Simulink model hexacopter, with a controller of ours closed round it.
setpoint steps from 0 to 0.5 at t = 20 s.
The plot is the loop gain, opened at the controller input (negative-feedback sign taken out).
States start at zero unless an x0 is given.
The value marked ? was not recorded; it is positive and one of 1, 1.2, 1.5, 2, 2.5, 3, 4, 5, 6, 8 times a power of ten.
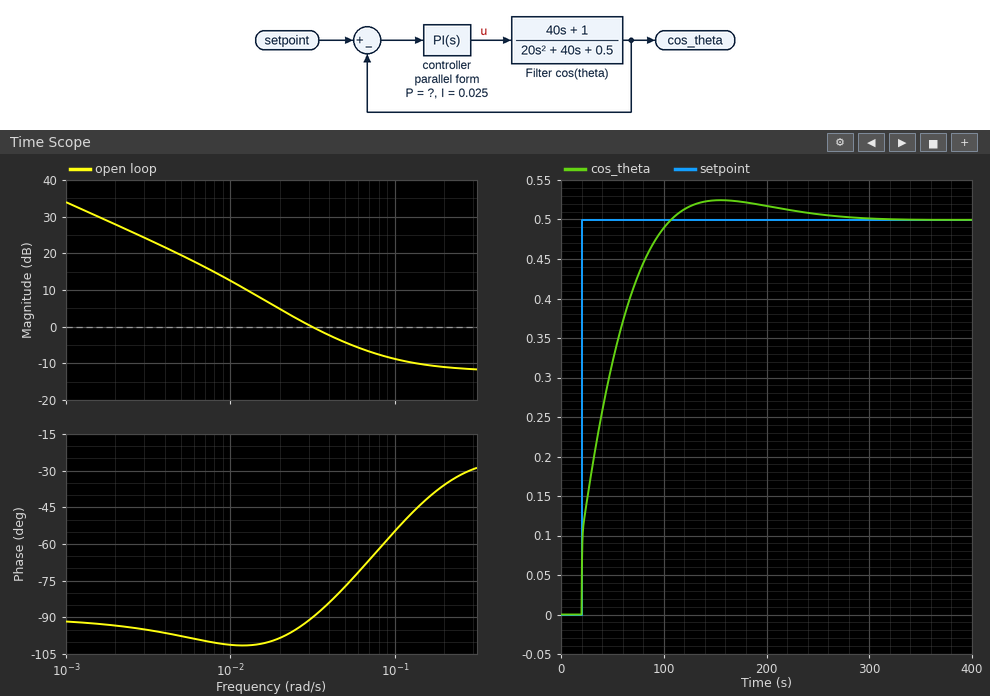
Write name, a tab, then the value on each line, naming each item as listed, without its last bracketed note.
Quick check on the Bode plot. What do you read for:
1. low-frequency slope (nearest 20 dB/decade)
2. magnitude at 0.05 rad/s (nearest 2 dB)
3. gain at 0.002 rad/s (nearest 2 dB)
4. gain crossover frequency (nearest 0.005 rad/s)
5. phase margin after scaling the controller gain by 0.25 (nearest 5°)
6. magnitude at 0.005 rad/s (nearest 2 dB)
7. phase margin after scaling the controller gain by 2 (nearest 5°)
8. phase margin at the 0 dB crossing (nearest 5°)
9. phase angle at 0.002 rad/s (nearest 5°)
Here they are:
low-frequency slope	-20 dB/decade
magnitude at 0.05 rad/s	-4 dB
gain at 0.002 rad/s	28 dB
gain crossover frequency	0.030 rad/s
phase margin after scaling the controller gain by 0.25	80°
magnitude at 0.005 rad/s	20 dB
phase margin after scaling the controller gain by 2	110°
phase margin at the 0 dB crossing	90°
phase angle at 0.002 rad/s	-95°
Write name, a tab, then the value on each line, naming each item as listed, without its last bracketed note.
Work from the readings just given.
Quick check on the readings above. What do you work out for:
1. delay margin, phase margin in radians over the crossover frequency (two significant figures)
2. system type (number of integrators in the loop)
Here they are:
delay margin, phase margin in radians over the crossover frequency	52 s
system type	1
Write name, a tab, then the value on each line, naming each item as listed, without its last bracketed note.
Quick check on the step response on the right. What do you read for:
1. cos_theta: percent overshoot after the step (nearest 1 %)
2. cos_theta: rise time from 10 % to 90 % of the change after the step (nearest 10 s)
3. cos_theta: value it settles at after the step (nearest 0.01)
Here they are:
cos_theta: percent overshoot after the step	5 %
cos_theta: rise time from 10 % to 90 % of the change after the step	60 s
cos_theta: value it settles at after the step	0.50
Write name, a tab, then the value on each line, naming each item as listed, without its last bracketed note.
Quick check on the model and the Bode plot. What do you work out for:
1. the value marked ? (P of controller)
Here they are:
the value marked ?	0.25
